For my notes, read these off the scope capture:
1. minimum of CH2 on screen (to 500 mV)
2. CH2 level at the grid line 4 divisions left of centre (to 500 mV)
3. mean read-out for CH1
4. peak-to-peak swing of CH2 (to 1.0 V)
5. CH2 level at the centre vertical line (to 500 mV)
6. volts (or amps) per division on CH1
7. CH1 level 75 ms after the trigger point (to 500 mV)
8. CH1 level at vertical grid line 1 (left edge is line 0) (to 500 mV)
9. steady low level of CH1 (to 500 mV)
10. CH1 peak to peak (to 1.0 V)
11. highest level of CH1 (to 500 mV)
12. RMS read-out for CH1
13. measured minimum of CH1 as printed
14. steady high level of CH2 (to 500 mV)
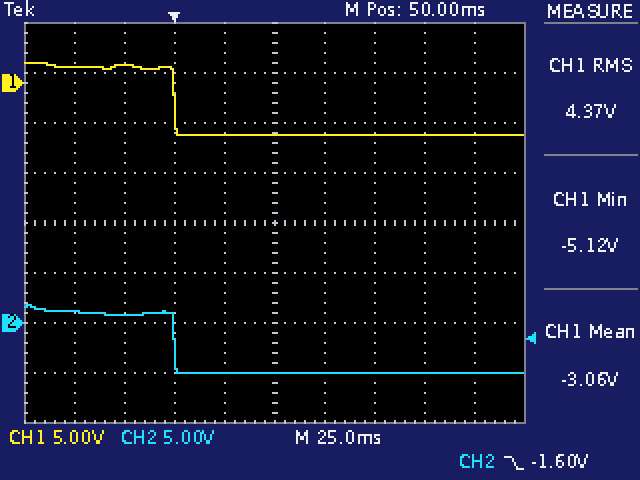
-5.0 V
1.0 V
-3.06 V
7.0 V
-5.0 V
5 V
-5.0 V
1.5 V
-5.0 V
7.0 V
2.0 V
4.37 V
-5.12 V
1.0 V
